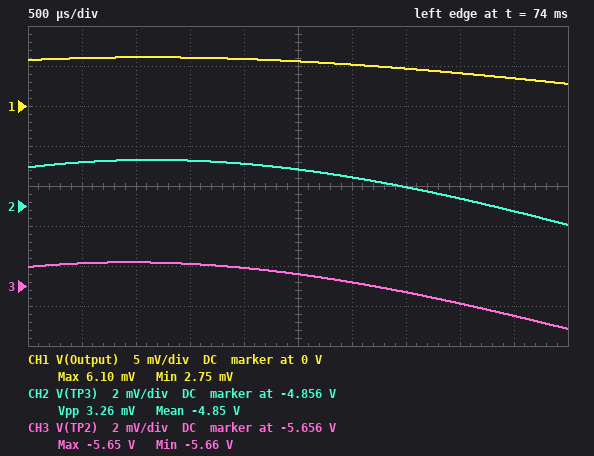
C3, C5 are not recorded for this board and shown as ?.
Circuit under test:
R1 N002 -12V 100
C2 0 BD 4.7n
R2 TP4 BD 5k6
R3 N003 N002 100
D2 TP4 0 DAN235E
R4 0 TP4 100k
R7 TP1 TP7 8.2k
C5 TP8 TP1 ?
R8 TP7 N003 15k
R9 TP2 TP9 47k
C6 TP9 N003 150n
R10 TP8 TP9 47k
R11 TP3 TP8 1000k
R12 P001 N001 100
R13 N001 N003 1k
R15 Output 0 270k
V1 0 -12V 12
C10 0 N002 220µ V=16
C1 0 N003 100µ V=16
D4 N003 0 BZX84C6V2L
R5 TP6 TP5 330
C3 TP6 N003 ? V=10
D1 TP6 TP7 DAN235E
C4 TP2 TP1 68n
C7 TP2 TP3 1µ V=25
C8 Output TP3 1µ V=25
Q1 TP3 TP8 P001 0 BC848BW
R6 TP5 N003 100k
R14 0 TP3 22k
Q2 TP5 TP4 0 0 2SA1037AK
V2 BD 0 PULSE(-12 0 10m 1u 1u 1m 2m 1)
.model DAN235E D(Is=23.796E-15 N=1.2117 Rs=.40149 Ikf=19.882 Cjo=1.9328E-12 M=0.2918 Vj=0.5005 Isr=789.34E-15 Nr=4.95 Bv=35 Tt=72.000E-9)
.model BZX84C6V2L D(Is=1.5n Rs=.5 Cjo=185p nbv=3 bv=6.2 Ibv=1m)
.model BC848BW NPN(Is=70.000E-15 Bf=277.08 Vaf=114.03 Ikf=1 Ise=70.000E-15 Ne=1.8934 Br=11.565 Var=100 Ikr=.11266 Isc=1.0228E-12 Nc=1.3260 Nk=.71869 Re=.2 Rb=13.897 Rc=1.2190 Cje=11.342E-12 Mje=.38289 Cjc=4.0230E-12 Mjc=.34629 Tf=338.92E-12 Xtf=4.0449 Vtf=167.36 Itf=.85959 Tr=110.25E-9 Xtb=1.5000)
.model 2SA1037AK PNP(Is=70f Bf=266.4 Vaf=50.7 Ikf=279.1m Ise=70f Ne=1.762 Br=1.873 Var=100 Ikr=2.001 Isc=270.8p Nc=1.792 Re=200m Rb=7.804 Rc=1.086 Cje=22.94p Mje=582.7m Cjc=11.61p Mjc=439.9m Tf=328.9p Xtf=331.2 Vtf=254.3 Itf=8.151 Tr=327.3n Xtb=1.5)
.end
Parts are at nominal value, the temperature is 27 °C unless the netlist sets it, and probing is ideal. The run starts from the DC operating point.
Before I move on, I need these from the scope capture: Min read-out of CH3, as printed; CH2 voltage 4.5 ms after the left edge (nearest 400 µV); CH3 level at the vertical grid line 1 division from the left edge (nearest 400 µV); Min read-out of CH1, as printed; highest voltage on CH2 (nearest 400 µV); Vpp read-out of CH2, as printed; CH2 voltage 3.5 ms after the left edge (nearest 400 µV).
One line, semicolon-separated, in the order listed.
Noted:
-5.66 V; -4.8564 V; -5.6548 V; 2.75 mV; -4.8536 V; 3.26 mV; -4.8552 V
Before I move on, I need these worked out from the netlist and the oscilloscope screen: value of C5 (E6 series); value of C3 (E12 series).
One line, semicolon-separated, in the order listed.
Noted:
150 nF; 8.2 µF
